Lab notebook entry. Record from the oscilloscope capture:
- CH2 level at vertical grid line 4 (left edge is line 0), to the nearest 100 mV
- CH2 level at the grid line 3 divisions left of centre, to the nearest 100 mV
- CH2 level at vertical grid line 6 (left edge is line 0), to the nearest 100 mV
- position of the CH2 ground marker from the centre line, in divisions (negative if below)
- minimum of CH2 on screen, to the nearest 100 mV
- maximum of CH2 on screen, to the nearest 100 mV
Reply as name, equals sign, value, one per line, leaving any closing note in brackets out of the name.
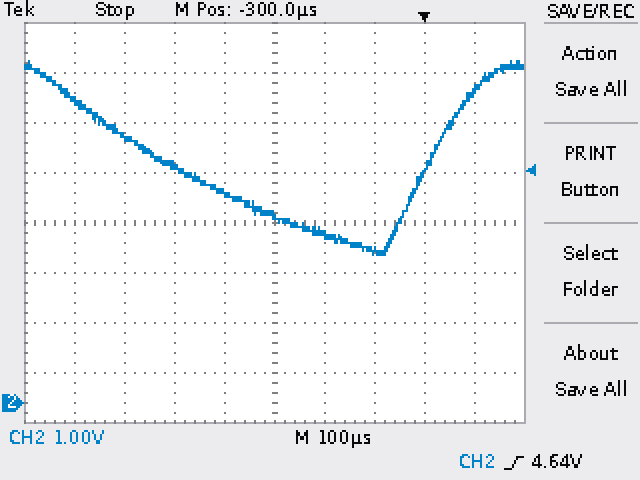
CH2 level at vertical grid line 4 (left edge is line 0), to the nearest 100 mV = 4.2 V
CH2 level at the grid line 3 divisions left of centre, to the nearest 100 mV = 5.3 V
CH2 level at vertical grid line 6 (left edge is line 0), to the nearest 100 mV = 3.4 V
position of the CH2 ground marker from the centre line, in divisions = -3.6 div
minimum of CH2 on screen, to the nearest 100 mV = 3.0 V
maximum of CH2 on screen, to the nearest 100 mV = 6.8 V
